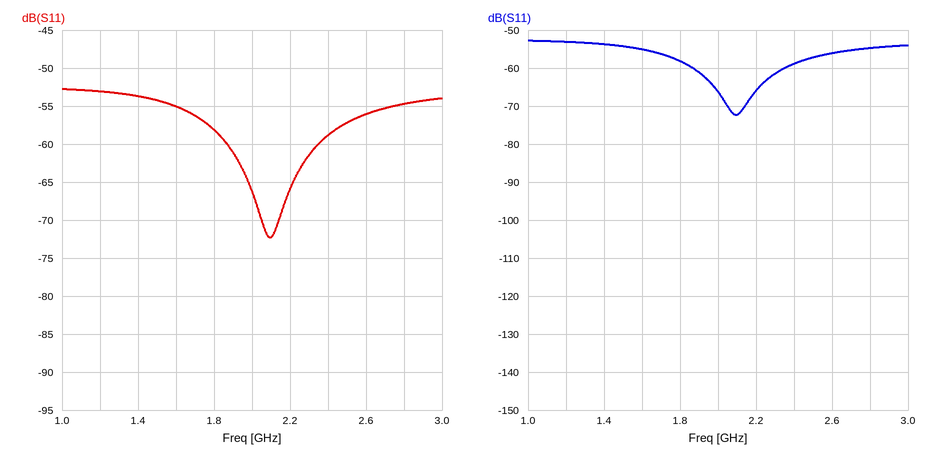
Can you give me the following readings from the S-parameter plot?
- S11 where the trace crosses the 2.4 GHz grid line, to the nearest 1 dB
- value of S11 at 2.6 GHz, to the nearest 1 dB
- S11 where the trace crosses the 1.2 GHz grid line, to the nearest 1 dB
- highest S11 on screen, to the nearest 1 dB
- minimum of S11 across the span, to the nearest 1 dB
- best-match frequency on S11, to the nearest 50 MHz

-59 dB
-56 dB
-53 dB
-53 dB
-72 dB
2.10 GHz
